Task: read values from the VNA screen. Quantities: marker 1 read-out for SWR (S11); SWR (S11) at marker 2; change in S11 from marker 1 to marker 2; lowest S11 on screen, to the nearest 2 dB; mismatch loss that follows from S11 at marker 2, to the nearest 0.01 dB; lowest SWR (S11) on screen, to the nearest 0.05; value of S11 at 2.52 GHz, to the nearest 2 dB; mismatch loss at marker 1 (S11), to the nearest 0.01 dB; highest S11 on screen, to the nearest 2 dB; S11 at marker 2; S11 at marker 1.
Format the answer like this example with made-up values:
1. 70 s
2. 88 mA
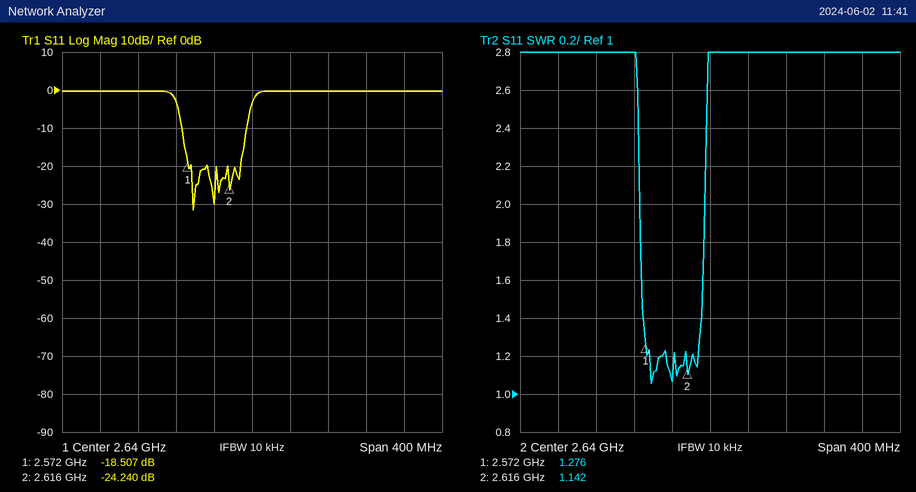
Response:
1. 1.276
2. 1.142
3. -5.733 dB
4. -32 dB
5. 0.02 dB
6. 1.05
7. 0 dB
8. 0.06 dB
9. 0 dB
10. -24.240 dB
11. -18.507 dB
